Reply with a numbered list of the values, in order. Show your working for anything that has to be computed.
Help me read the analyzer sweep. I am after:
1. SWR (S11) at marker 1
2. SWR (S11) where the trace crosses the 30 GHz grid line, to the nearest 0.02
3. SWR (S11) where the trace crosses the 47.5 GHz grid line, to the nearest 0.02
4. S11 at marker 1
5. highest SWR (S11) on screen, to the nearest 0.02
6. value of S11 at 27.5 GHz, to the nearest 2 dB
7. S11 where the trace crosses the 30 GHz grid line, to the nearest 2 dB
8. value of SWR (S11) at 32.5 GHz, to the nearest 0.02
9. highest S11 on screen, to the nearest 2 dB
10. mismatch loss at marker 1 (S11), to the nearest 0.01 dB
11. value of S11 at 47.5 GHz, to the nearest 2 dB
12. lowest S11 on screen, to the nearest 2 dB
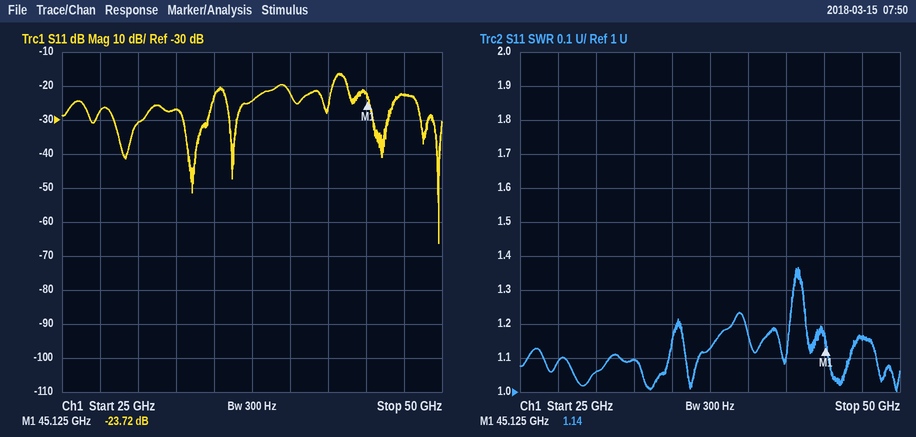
1. 1.14
2. 1.06
3. 1.16
4. -23.72 dB
5. 1.36
6. -28 dB
7. -30 dB
8. 1.10
9. -16 dB
10. −10 log10(1 − 10^(-23.72/10)) ≈ 0.02 dB
11. -22 dB
12. -66 dB
